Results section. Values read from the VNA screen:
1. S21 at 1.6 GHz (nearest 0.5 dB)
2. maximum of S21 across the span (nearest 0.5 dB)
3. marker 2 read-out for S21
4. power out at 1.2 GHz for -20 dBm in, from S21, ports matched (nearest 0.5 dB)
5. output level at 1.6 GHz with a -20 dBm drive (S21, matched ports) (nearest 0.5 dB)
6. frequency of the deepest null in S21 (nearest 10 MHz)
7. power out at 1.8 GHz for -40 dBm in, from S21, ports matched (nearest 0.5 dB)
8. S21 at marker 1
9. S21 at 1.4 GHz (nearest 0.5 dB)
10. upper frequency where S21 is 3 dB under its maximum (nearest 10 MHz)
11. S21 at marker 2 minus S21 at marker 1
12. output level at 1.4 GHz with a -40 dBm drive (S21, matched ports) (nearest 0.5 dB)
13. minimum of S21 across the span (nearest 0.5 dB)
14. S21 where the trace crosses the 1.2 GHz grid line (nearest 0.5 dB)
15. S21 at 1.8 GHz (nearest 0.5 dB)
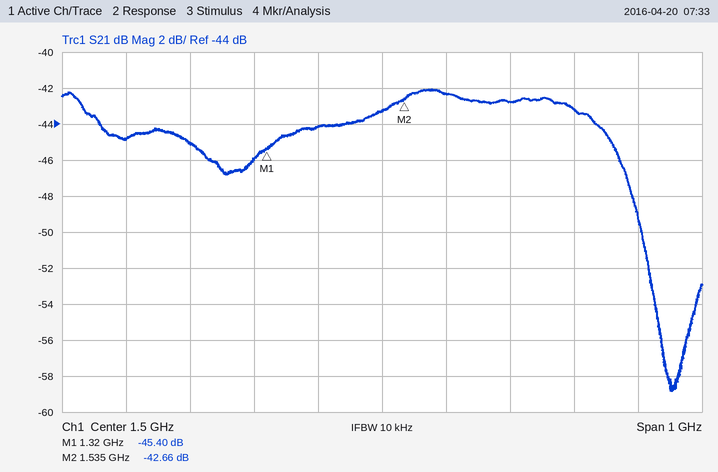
-42.5 dB
-42.0 dB
-42.66 dB
-65.0 dBm
-62.5 dBm
1.95 GHz
-83.0 dBm
-45.40 dB
-44.0 dB
1.86 GHz
2.74 dB
-84.0 dBm
-59.0 dB
-45.0 dB
-43.0 dB
